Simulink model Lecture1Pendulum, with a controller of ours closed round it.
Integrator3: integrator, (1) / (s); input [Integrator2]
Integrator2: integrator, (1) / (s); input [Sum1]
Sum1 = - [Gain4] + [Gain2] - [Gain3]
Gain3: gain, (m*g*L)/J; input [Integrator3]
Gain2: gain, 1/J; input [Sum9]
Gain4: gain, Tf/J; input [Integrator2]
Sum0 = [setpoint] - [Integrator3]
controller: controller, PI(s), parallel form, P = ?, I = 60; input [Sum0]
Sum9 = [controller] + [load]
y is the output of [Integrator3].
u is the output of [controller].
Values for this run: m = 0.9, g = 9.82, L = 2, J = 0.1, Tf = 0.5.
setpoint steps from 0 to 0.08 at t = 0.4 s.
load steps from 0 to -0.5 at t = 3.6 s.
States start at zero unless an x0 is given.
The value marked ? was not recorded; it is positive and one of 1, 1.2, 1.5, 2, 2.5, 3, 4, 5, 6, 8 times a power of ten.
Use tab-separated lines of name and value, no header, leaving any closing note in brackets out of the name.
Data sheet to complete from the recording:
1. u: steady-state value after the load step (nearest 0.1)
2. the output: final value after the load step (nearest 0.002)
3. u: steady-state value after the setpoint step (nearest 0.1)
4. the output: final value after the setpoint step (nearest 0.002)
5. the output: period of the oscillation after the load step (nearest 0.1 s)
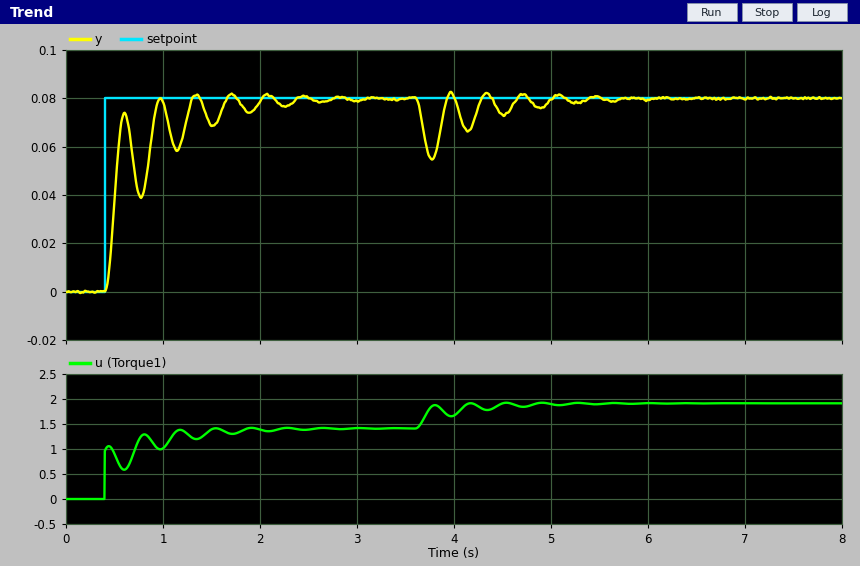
u: steady-state value after the load step	1.9
the output: final value after the load step	0.080
u: steady-state value after the setpoint step	1.4
the output: final value after the setpoint step	0.080
the output: period of the oscillation after the load step	0.4 s
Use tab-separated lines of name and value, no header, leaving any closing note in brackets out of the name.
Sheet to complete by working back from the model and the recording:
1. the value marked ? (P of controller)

the value marked ?	12
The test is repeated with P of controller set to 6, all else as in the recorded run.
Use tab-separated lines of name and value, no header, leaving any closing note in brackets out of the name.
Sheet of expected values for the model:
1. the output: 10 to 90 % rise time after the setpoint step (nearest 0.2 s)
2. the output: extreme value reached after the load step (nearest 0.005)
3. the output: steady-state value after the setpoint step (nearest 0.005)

the output: 10 to 90 % rise time after the setpoint step	0.6 s
the output: extreme value reached after the load step	0.050
the output: steady-state value after the setpoint step	0.080
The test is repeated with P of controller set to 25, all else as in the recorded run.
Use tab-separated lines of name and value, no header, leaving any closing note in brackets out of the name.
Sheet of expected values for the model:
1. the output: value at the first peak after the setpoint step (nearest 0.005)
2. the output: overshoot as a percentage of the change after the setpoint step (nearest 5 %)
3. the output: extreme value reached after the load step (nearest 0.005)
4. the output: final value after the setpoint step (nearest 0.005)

the output: value at the first peak after the setpoint step	0.090
the output: overshoot as a percentage of the change after the setpoint step	10 %
the output: extreme value reached after the load step	0.060
the output: final value after the setpoint step	0.080
